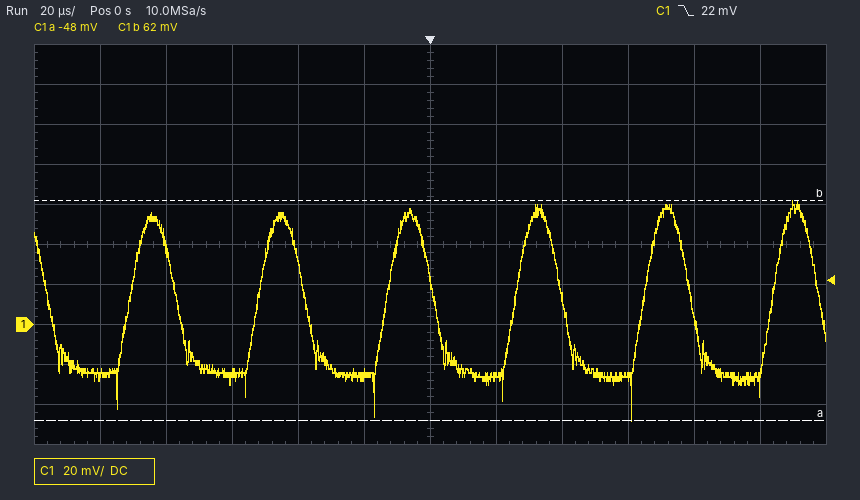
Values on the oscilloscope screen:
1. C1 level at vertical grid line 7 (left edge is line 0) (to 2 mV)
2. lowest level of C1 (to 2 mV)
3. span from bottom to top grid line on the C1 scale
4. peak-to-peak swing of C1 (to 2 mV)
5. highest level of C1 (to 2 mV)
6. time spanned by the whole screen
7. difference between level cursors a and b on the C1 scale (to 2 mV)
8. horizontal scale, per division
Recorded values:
-26 mV
-48 mV
200 mV
110 mV
62 mV
240 µs
110 mV
20 µs
